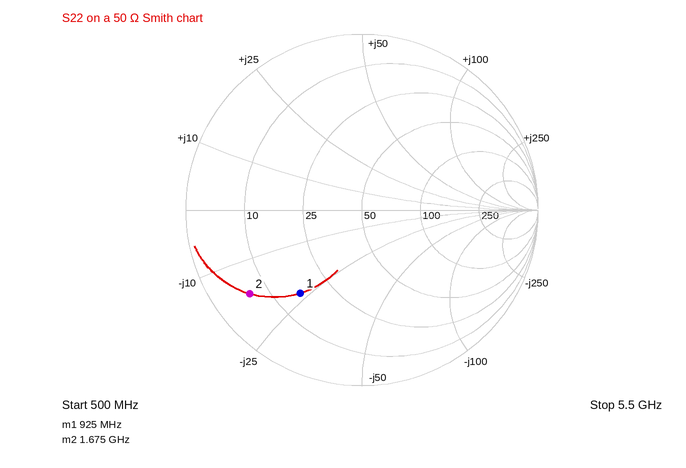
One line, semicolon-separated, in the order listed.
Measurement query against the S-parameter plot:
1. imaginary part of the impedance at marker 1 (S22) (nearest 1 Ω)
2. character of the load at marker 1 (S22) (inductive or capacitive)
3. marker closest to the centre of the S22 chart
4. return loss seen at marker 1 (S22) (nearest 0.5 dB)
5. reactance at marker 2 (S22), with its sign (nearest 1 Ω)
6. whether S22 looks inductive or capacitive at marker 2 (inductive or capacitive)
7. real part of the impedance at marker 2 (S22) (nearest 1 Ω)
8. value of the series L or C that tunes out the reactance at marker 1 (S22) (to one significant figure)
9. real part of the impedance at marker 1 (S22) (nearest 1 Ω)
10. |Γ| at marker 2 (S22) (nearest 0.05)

-23 Ω; capacitive; marker 1; 4.5 dB; -16 Ω; capacitive; 6 Ω; 4 nH; 16 Ω; 0.80
